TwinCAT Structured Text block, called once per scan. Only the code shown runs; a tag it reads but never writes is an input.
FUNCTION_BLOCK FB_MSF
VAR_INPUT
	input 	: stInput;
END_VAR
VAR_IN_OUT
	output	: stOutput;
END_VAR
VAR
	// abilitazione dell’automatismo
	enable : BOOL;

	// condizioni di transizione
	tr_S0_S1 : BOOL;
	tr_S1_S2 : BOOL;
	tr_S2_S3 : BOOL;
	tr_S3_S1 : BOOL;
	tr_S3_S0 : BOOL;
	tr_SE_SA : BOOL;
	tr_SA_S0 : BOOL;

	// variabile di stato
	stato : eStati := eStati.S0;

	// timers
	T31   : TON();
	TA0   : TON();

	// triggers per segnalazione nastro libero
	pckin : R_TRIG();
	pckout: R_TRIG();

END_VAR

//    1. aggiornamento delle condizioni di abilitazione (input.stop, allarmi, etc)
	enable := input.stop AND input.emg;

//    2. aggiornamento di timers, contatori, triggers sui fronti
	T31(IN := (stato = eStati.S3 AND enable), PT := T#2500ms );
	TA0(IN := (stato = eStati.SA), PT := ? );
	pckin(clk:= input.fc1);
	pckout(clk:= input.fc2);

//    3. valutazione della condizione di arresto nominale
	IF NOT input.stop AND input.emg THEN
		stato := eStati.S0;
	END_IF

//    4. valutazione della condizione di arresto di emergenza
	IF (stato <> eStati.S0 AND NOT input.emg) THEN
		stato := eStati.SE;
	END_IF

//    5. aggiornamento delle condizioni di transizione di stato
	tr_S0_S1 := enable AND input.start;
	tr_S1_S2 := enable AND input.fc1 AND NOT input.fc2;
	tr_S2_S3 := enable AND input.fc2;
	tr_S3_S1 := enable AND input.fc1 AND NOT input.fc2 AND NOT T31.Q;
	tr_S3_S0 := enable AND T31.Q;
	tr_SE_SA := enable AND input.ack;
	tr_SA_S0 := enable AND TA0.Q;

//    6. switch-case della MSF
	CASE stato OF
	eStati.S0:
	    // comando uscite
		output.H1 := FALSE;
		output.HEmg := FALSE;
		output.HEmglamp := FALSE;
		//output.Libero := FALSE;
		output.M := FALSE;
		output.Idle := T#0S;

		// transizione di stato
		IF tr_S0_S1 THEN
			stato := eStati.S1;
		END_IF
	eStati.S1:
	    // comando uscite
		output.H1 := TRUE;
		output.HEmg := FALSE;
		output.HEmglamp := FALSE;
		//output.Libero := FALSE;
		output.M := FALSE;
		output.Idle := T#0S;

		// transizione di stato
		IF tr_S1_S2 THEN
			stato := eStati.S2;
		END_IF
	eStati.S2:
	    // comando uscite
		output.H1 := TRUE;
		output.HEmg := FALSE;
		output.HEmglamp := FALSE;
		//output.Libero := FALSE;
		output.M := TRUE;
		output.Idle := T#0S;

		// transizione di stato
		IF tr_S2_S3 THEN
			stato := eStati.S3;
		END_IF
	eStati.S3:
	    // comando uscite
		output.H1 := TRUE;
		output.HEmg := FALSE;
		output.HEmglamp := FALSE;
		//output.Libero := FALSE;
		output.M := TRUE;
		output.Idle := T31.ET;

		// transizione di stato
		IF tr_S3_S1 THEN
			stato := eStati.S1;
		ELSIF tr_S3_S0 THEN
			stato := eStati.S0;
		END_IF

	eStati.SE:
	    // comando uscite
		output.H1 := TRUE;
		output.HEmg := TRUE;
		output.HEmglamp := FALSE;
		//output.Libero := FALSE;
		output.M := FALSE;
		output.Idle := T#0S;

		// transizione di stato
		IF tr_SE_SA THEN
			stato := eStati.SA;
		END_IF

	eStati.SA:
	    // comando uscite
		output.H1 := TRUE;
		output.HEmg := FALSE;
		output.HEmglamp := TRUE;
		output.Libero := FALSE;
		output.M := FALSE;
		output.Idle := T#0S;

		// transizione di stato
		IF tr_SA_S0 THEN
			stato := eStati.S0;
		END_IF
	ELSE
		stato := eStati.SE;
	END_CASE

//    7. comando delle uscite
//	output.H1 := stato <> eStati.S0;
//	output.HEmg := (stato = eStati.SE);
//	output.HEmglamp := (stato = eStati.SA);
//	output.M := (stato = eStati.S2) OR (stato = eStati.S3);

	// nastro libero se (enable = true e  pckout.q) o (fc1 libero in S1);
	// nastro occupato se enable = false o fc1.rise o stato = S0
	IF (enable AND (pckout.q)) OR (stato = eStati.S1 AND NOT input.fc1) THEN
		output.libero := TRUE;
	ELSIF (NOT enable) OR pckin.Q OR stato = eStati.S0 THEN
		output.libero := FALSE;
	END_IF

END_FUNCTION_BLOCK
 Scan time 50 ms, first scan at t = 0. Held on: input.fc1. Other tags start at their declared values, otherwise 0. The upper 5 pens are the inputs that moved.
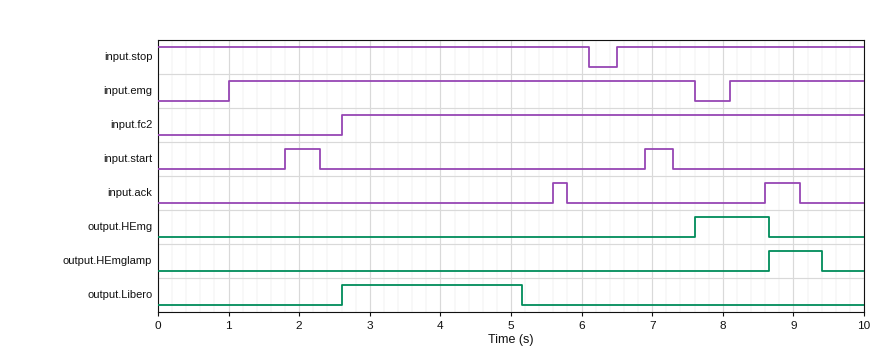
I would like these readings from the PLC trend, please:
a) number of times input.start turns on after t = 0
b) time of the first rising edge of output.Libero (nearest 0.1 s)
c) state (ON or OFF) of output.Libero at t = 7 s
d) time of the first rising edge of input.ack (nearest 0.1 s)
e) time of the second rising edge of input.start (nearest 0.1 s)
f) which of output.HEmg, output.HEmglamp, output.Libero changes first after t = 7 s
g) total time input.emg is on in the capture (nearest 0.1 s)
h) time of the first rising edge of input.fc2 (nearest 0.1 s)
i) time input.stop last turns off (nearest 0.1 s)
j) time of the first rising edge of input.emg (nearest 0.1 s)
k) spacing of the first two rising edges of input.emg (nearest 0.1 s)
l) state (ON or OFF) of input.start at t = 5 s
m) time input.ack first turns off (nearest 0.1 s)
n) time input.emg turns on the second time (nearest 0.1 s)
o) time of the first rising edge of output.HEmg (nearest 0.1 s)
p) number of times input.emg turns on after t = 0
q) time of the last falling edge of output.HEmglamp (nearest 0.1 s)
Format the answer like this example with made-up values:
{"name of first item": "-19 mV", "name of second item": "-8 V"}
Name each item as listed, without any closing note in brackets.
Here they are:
{"number of times input.start turns on after t = 0": "2", "time of the first rising edge of output.Libero": "2.6 s", "state (ON or OFF) of output.Libero at t = 7 s": "OFF", "time of the first rising edge of input.ack": "5.6 s", "time of the second rising edge of input.start": "6.9 s", "which of output.HEmg, output.HEmglamp, output.Libero changes first after t = 7 s": "output.HEmg", "total time input.emg is on in the capture": "8.5 s", "time of the first rising edge of input.fc2": "2.6 s", "time input.stop last turns off": "6.1 s", "time of the first rising edge of input.emg": "1.0 s", "spacing of the first two rising edges of input.emg": "7.1 s", "state (ON or OFF) of input.start at t = 5 s": "OFF", "time input.ack first turns off": "5.8 s", "time input.emg turns on the second time": "8.1 s", "time of the first rising edge of output.HEmg": "7.6 s", "number of times input.emg turns on after t = 0": "2", "time of the last falling edge of output.HEmglamp": "9.4 s"}
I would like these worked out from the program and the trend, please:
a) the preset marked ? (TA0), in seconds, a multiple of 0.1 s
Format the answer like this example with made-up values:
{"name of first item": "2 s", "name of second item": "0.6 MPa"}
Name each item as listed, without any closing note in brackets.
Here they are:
{"the preset marked ? (TA0), in seconds, a multiple of 0.1 s": "0.7 s"}
